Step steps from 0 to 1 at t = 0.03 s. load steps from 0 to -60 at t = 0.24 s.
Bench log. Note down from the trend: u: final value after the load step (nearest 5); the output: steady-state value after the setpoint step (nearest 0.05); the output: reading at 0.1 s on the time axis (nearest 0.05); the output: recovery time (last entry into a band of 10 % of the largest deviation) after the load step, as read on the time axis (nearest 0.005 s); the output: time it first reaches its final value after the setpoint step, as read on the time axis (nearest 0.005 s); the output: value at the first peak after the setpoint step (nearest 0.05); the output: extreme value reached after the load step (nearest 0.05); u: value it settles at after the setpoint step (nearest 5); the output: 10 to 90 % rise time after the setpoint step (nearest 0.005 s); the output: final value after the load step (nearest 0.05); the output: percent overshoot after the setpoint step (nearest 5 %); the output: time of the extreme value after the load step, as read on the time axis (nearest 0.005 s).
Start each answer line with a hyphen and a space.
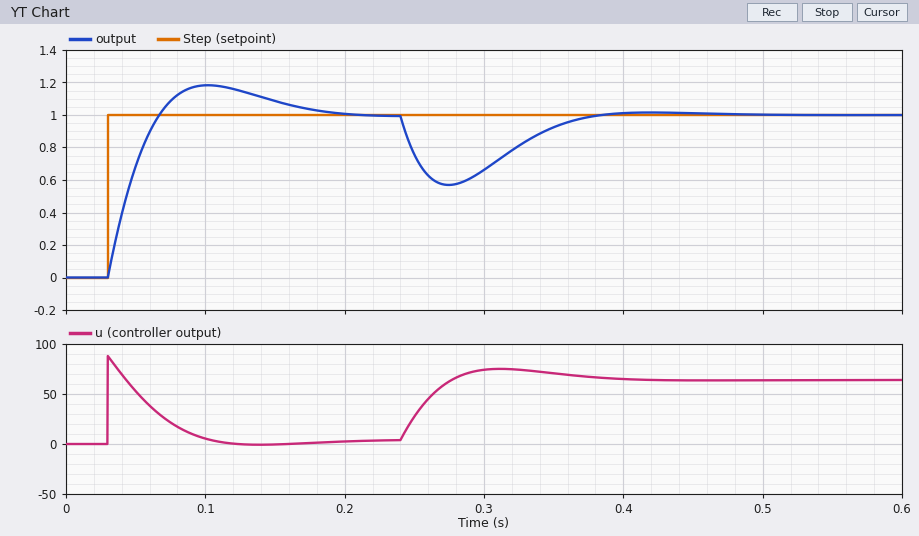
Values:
- 65
- 1.00
- 1.20
- 0.360 s
- 0.065 s
- 1.20
- 0.55
- 5
- 0.030 s
- 1.00
- 20 %
- 0.275 s
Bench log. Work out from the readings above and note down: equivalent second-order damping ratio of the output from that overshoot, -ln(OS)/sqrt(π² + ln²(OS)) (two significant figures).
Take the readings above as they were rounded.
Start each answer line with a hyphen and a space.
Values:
- 0.46
